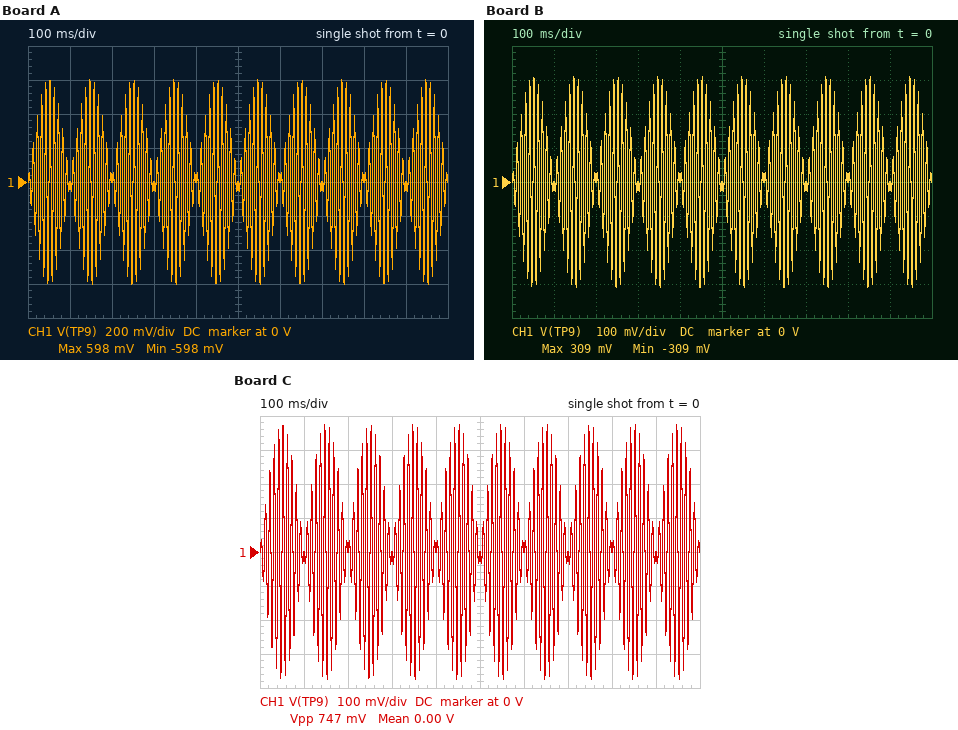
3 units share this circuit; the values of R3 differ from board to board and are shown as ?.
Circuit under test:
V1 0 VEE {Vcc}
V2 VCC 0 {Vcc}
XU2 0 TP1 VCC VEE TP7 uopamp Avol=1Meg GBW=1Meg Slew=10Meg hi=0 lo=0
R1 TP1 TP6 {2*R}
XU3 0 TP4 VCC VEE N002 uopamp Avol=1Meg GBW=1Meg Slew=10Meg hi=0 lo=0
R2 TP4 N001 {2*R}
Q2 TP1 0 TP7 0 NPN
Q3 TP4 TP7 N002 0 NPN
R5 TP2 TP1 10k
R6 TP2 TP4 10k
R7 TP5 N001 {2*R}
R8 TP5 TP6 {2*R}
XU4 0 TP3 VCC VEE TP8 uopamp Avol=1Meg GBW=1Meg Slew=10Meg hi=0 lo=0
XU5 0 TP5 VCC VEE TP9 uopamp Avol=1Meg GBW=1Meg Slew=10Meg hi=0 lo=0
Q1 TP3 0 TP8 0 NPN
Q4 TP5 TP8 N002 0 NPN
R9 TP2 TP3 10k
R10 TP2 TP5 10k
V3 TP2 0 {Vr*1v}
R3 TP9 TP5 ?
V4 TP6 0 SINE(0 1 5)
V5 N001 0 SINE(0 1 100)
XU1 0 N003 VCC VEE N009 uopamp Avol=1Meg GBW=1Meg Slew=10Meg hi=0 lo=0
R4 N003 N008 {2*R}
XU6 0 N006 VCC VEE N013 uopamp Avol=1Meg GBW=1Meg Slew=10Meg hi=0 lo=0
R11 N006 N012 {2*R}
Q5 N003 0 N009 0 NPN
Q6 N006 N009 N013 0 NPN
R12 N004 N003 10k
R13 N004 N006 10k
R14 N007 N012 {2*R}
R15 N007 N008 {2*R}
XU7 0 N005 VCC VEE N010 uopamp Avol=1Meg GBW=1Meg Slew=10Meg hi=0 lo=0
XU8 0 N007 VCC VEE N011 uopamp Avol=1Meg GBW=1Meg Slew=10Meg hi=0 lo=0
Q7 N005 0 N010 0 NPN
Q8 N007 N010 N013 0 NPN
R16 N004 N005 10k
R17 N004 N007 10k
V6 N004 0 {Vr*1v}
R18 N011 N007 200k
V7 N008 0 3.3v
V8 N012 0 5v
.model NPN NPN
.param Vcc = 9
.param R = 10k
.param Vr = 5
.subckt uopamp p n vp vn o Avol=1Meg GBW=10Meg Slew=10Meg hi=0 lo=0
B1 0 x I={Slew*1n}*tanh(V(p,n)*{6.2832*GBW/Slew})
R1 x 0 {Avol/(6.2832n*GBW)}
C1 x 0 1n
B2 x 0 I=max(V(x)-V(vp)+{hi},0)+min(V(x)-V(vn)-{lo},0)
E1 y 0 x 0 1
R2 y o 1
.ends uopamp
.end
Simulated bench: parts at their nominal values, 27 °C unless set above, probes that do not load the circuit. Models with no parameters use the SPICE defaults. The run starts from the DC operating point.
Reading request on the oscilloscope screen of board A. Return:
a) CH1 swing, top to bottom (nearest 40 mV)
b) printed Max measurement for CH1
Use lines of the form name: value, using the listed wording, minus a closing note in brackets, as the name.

CH1 swing, top to bottom: 1.20 V
printed Max measurement for CH1: 598 mV
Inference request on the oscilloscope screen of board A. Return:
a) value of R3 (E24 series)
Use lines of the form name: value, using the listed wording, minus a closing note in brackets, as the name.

value of R3: 120 kΩ
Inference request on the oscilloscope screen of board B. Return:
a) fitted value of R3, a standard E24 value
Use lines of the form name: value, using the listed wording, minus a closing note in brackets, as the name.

fitted value of R3, a standard E24 value: 62 kΩ
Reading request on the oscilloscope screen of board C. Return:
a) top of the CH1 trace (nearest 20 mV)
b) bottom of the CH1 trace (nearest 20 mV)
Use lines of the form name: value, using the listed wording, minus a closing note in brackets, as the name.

top of the CH1 trace: 380 mV
bottom of the CH1 trace: -380 mV
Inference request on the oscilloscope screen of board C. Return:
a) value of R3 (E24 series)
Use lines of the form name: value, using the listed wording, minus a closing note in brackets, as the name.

value of R3: 75 kΩ
